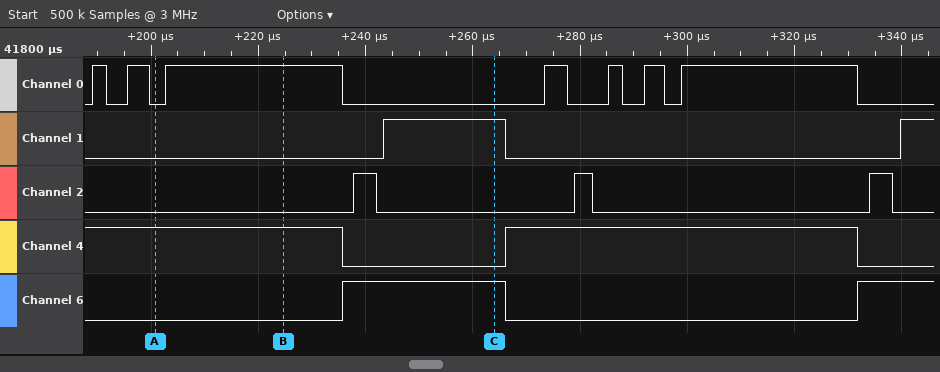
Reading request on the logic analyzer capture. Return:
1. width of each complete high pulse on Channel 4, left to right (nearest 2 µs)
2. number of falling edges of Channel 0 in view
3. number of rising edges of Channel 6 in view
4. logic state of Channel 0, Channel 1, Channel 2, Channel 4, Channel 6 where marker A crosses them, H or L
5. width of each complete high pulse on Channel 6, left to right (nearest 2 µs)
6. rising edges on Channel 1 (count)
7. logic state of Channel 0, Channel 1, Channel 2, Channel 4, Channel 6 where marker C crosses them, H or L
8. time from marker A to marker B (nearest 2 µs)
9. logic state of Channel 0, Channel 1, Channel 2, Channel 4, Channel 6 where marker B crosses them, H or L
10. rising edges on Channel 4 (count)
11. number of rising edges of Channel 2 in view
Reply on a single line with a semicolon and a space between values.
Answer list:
66 µs; 7; 2; Channel 0=L, Channel 1=L, Channel 2=L, Channel 4=H, Channel 6=L; 30 µs; 2; Channel 0=L, Channel 1=H, Channel 2=L, Channel 4=L, Channel 6=H; 24 µs; Channel 0=H, Channel 1=L, Channel 2=L, Channel 4=H, Channel 6=L; 1; 3
